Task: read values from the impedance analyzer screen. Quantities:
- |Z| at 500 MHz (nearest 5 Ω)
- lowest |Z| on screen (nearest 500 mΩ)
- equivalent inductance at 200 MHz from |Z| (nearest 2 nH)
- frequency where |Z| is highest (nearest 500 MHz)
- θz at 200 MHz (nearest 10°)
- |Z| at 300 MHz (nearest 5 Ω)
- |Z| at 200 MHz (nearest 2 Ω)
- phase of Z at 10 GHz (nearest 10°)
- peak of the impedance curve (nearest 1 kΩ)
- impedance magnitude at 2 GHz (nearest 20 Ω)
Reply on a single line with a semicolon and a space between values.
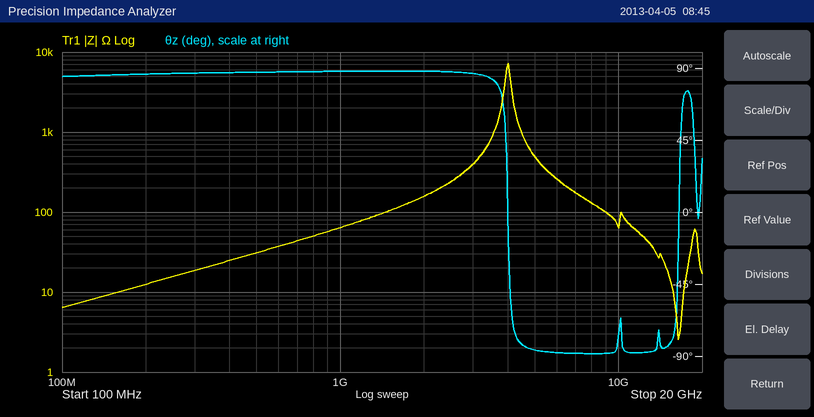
30 Ω; 2.5 Ω; 10 nH; 4.0 GHz; 90°; 20 Ω; 12 Ω; -80°; 7 kΩ; 160 Ω
